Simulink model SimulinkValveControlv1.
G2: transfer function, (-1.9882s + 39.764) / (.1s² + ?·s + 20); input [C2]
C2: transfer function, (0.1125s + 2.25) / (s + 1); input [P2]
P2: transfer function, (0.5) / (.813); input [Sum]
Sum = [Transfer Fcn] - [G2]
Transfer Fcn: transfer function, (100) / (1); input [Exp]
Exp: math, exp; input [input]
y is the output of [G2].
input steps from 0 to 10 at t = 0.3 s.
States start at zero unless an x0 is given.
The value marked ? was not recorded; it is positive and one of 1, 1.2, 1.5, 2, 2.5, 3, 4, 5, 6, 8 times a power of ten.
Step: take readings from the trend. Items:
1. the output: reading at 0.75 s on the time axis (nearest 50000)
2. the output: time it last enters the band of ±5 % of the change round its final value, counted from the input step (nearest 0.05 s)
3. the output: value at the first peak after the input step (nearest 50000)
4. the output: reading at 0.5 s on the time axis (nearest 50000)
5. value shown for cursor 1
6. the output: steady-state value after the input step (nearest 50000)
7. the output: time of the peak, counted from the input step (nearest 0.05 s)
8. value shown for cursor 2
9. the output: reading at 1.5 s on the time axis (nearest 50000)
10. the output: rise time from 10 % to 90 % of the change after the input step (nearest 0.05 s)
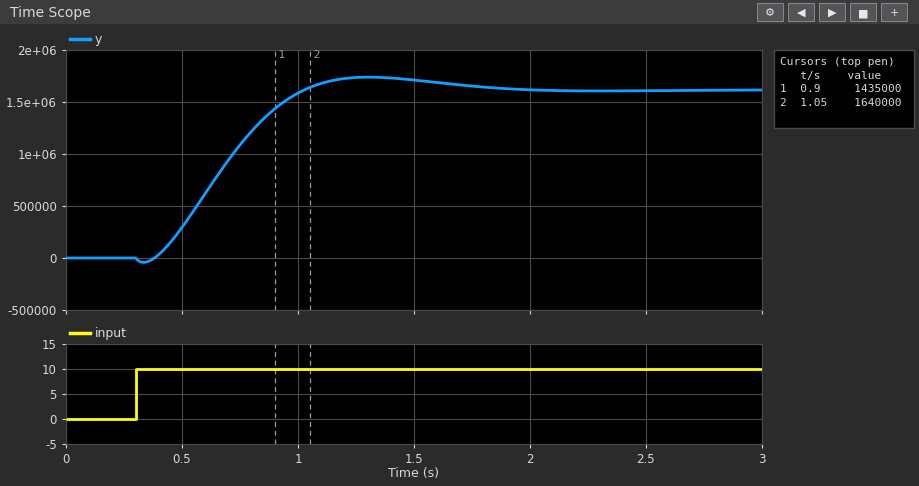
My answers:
1100000
1.25 s
1750000
300000
1435000
1600000
1.00 s
1640000
1700000
0.45 s
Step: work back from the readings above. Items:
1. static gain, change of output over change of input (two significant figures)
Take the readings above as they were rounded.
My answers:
160000
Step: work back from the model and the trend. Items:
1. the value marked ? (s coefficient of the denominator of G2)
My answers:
5
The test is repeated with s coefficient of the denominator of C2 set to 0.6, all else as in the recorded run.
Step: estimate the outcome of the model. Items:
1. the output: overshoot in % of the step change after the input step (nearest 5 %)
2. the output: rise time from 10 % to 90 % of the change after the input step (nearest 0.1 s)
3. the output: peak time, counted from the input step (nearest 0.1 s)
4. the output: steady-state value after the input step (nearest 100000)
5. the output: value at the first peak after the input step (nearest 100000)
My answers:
15 %
0.3 s
0.7 s
1600000
1800000
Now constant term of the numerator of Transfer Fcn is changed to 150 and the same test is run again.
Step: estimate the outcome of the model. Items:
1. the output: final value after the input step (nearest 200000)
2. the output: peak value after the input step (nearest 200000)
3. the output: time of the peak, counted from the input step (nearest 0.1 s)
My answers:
2400000
2600000
1.0 s
